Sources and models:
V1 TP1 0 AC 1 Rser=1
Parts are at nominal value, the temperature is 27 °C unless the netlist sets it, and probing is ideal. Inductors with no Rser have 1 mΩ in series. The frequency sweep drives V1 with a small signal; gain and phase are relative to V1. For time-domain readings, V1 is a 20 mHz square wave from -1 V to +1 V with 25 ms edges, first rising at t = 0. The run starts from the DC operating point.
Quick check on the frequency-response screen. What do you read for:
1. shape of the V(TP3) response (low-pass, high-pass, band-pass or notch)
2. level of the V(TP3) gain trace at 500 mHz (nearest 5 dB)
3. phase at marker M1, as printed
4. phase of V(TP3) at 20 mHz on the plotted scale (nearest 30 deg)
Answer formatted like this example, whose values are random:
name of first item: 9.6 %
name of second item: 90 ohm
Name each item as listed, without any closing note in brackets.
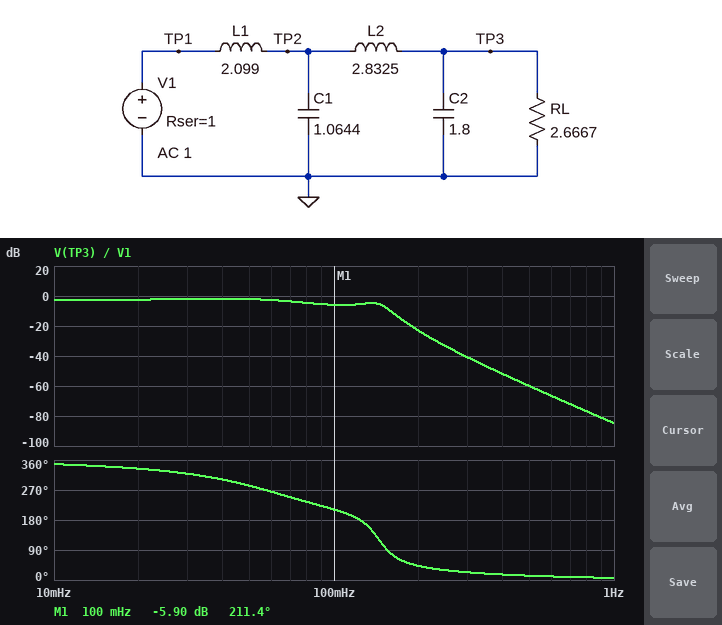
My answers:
shape of the V(TP3) response: low-pass
level of the V(TP3) gain trace at 500 mHz: -60 dB
phase at marker M1, as printed: 211.4 deg
phase of V(TP3) at 20 mHz on the plotted scale: 330 deg
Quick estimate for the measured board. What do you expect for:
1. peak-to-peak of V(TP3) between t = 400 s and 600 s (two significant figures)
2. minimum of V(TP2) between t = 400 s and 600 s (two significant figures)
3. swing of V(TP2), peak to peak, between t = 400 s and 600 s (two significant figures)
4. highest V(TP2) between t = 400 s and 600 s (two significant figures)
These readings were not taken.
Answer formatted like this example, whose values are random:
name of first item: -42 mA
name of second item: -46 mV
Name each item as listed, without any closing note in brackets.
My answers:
peak-to-peak of V(TP3) between t = 400 s and 600 s: 1.8 V
minimum of V(TP2) between t = 400 s and 600 s: -1.1 V
swing of V(TP2), peak to peak, between t = 400 s and 600 s: 2.2 V
highest V(TP2) between t = 400 s and 600 s: 1.1 V
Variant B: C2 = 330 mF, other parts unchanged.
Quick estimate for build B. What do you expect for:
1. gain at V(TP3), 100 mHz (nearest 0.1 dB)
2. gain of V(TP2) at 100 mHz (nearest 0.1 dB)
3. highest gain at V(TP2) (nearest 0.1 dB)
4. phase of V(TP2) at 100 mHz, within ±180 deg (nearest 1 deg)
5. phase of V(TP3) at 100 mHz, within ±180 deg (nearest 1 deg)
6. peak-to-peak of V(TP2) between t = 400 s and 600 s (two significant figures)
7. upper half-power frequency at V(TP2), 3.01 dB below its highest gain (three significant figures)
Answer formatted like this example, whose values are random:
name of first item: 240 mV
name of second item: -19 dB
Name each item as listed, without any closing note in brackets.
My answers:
gain at V(TP3), 100 mHz: -1.8 dB
gain of V(TP2) at 100 mHz: -2.6 dB
highest gain at V(TP2): -2.4 dB
phase of V(TP2) at 100 mHz, within ±180 deg: -56 deg
phase of V(TP3) at 100 mHz, within ±180 deg: -103 deg
peak-to-peak of V(TP2) between t = 400 s and 600 s: 1.8 V
upper half-power frequency at V(TP2), 3.01 dB below its highest gain: 192 mHz
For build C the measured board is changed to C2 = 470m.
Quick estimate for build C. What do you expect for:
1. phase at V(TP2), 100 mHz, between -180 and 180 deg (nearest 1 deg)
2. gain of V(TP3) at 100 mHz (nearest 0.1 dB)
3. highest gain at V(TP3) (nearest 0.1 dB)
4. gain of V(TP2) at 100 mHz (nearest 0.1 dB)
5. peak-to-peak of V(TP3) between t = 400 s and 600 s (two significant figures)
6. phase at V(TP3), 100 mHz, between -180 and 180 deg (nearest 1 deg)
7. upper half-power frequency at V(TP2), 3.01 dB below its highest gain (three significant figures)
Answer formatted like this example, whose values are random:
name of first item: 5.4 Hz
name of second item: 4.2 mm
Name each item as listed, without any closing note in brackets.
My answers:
phase at V(TP2), 100 mHz, between -180 and 180 deg: -54 deg
gain of V(TP3) at 100 mHz: -2.0 dB
highest gain at V(TP3): -1.8 dB
gain of V(TP2) at 100 mHz: -3.7 dB
peak-to-peak of V(TP3) between t = 400 s and 600 s: 2.1 V
phase at V(TP3), 100 mHz, between -180 and 180 deg: -109 deg
upper half-power frequency at V(TP2), 3.01 dB below its highest gain: 196 mHz
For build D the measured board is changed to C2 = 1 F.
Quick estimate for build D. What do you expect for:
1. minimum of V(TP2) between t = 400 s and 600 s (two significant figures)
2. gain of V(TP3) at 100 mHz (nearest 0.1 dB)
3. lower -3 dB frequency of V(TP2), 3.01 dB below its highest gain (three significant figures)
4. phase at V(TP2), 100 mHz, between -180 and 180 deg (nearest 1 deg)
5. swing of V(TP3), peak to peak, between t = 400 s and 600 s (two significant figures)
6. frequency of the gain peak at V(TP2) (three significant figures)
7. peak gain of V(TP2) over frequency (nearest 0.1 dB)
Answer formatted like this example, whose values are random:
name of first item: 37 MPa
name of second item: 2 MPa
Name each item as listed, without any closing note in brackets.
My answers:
minimum of V(TP2) between t = 400 s and 600 s: -1.0 V
gain of V(TP3) at 100 mHz: -3.2 dB
lower -3 dB frequency of V(TP2), 3.01 dB below its highest gain: 133 mHz
phase at V(TP2), 100 mHz, between -180 and 180 deg: -29 deg
swing of V(TP3), peak to peak, between t = 400 s and 600 s: 2.0 V
frequency of the gain peak at V(TP2): 152 mHz
peak gain of V(TP2) over frequency: 3.0 dB
